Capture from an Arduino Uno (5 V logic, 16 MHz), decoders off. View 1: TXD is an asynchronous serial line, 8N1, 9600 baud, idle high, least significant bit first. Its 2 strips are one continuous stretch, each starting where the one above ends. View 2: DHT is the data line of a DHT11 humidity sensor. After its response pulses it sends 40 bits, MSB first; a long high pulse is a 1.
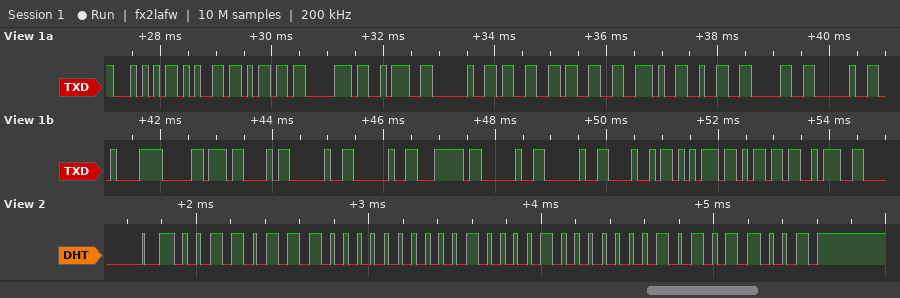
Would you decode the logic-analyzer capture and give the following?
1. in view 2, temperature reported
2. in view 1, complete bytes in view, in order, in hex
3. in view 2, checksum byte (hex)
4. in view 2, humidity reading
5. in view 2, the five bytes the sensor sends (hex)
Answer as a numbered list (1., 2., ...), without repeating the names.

1. 33.1 °C
2. 54 65 6D 70 3A 20 33 33 2E 32 30 20 C2 B0 43 20 20 7C 20 20 48 75 6D 3A
3. 0x59
4. 55 %
5. 37 00 21 01 59
